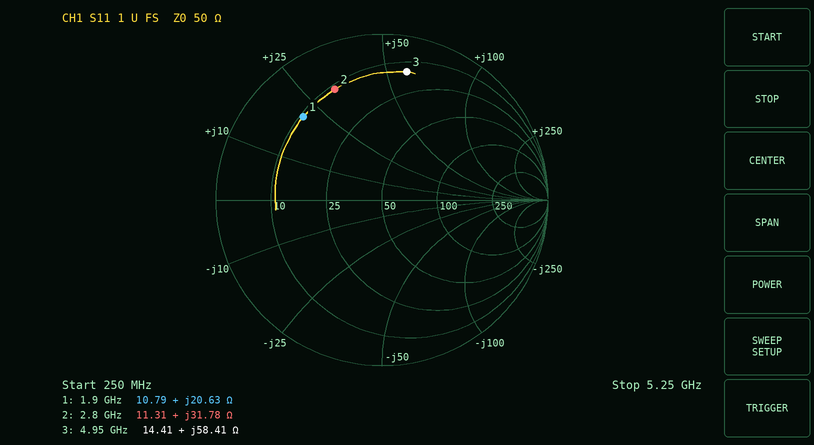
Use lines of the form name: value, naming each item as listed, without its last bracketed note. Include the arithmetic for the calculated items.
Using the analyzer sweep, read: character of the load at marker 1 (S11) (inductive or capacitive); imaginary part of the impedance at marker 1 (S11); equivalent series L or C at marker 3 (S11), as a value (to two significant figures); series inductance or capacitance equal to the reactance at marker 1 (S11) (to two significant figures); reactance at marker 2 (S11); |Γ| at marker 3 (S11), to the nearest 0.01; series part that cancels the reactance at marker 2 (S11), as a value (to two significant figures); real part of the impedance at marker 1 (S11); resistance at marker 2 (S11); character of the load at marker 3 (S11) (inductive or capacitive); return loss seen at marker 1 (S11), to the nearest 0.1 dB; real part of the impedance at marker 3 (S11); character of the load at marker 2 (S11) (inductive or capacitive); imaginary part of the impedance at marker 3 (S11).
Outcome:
character of the load at marker 1 (S11): inductive
imaginary part of the impedance at marker 1: +20.63 Ω
equivalent series L or C at marker 3 (S11), as a value: L = 58.41 Ω/(2π × 4.95 GHz) ≈ 1.9 nH
series inductance or capacitance equal to the reactance at marker 1 (S11): L = 20.63 Ω/(2π × 1.9 GHz) ≈ 1.7 nH
reactance at marker 2: +31.78 Ω
|Γ| at marker 3 (S11), to the nearest 0.01: 0.79
series part that cancels the reactance at marker 2 (S11), as a value: C = 1/(2π × 2.8 GHz × 31.78 Ω) ≈ 1.8 pF
real part of the impedance at marker 1: 10.79 Ω
resistance at marker 2: 11.31 Ω
character of the load at marker 3 (S11): inductive
return loss seen at marker 1 (S11), to the nearest 0.1 dB: 3.2 dB
real part of the impedance at marker 3: 14.41 Ω
character of the load at marker 2 (S11): inductive
imaginary part of the impedance at marker 3: +58.41 Ω
